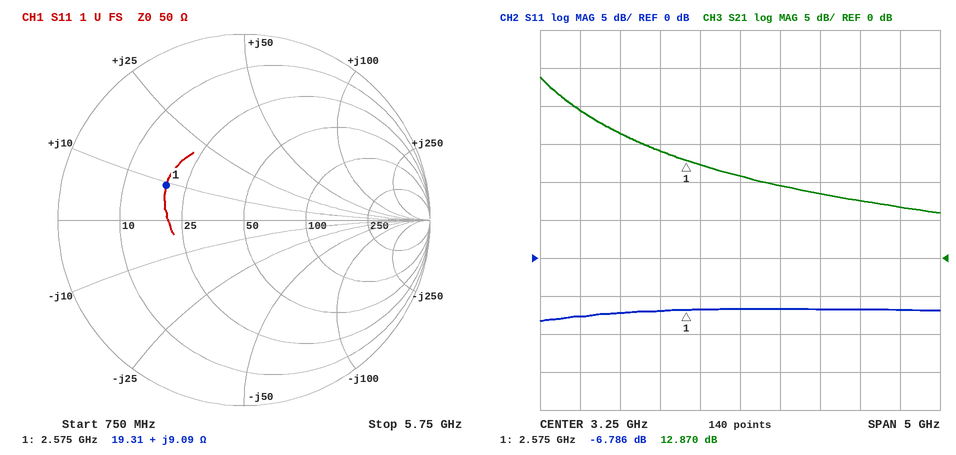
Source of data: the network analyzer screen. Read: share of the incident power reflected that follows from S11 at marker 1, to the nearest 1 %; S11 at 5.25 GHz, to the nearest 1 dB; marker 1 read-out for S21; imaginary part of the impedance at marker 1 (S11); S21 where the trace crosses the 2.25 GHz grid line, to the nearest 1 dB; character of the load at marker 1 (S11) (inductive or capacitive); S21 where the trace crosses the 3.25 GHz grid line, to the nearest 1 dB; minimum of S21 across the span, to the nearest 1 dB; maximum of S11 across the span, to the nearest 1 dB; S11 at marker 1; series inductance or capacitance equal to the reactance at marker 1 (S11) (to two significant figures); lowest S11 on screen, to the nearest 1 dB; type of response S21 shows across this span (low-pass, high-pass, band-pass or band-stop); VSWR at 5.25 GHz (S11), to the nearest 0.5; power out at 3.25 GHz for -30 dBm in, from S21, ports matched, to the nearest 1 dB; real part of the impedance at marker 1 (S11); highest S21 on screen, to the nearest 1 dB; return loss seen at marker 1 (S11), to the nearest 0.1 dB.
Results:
21 %
-7 dB
12.870 dB
+9.09 Ω
14 dB
inductive
11 dB
6 dB
-7 dB
-6.786 dB
560 pH
-8 dB
low-pass
2.5
-19 dBm
19.31 Ω
24 dB
6.8 dB
